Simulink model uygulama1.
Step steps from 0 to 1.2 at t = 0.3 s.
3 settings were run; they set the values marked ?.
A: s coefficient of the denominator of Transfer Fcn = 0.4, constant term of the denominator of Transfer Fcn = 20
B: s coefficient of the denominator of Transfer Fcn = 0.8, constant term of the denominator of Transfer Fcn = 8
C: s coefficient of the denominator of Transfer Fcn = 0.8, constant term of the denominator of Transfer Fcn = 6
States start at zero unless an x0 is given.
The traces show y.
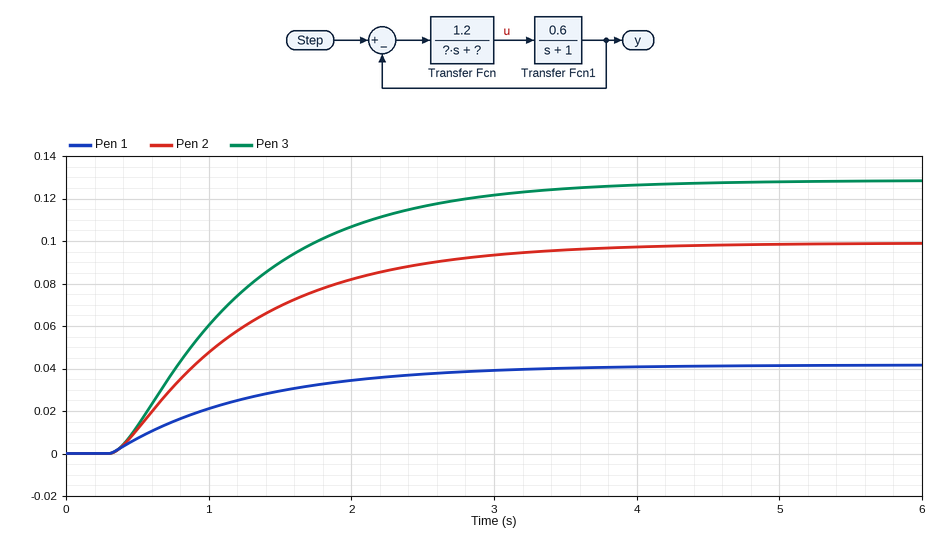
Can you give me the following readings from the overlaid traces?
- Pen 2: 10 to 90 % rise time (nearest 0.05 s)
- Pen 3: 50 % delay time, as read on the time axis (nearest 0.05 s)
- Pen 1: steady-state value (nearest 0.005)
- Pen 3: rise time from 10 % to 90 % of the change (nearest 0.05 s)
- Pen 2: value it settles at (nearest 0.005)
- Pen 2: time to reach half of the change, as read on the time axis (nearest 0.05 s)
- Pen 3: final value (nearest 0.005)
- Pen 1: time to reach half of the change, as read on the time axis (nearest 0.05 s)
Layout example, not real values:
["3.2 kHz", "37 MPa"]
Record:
["2.00 s", "1.05 s", "0.040", "1.95 s", "0.100", "1.05 s", "0.130", "1.00 s"]
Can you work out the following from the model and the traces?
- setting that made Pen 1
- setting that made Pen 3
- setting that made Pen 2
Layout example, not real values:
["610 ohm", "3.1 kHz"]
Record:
["A", "C", "B"]
